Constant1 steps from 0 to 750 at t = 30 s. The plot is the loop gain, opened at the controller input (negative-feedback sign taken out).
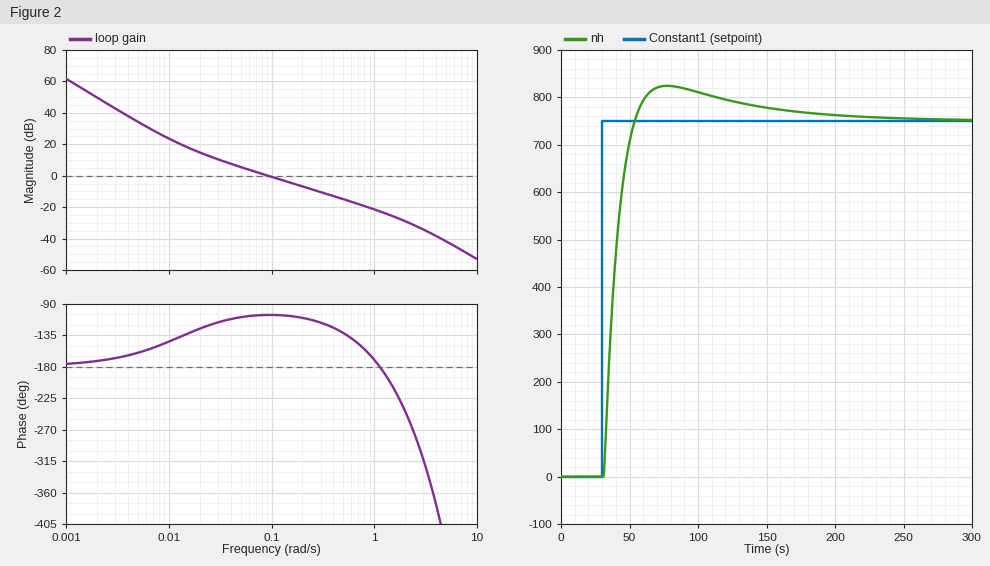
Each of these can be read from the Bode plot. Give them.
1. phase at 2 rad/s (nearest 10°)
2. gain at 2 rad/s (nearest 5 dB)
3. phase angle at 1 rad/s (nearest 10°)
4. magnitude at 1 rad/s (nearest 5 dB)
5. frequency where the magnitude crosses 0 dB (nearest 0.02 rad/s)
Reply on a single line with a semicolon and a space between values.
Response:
-240°; -30 dB; -170°; -20 dB; 0.10 rad/s
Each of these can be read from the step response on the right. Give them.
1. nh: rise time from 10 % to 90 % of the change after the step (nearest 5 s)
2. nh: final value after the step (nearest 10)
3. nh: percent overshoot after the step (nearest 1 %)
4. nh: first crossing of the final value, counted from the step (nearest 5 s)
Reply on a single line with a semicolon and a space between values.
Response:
15 s; 750; 10 %; 25 s
